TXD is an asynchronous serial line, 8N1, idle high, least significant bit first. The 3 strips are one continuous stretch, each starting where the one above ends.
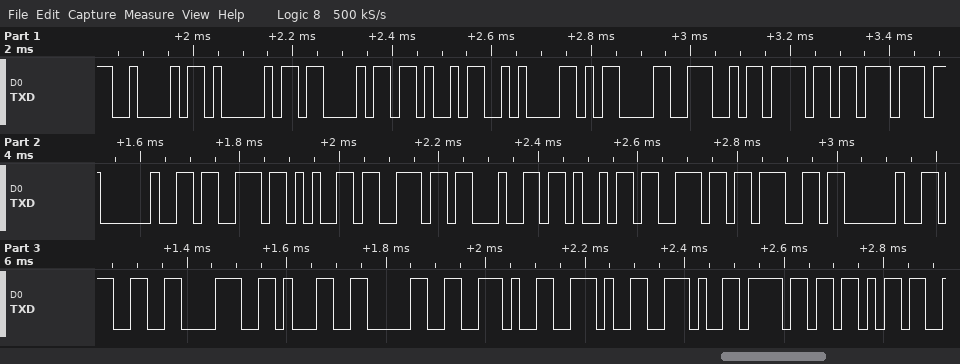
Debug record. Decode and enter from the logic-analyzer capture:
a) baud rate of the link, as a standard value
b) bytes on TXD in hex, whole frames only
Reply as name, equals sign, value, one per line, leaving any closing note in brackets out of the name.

baud rate of the link, as a standard value = 57600 baud
bytes on TXD in hex, whole frames only = 42 41 43 4B 0A 0D 4E 6F 77 20 73 65 6E 64 69 6E 67 20 33 38 31 30 2E 2E 2E 6F 6B
